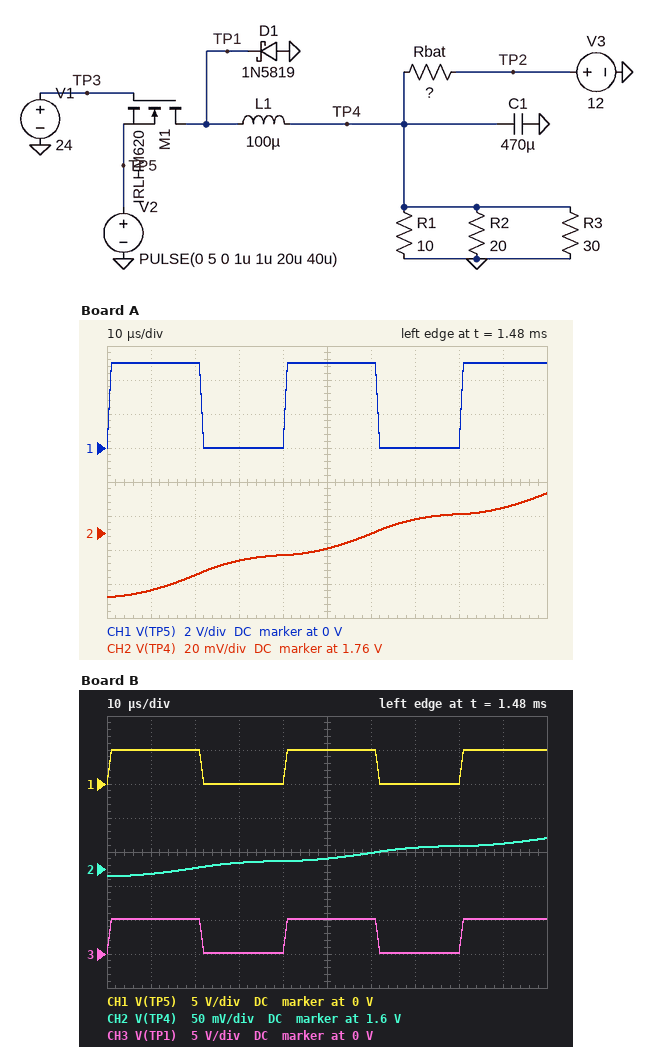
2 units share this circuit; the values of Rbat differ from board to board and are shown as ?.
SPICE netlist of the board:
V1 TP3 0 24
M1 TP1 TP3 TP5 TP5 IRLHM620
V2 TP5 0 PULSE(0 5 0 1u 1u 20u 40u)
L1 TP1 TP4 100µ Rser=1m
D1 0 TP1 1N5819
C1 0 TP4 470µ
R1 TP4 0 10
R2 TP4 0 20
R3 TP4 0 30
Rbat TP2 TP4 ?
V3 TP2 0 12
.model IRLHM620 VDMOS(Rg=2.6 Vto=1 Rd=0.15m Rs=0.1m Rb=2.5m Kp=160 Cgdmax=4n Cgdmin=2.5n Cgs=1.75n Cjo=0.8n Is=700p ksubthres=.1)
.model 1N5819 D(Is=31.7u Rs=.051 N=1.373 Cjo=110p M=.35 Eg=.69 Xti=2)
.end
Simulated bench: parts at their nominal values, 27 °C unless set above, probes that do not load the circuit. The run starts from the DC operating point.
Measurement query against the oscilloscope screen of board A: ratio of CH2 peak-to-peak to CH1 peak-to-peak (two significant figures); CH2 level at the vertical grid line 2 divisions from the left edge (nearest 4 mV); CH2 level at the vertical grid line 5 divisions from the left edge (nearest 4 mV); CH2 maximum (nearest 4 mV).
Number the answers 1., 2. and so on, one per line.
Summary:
1. 0.012
2. 1.736 V
3. 1.752 V
4. 1.784 V
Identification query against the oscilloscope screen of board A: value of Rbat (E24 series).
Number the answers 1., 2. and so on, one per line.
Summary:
1. 0.051 Ω
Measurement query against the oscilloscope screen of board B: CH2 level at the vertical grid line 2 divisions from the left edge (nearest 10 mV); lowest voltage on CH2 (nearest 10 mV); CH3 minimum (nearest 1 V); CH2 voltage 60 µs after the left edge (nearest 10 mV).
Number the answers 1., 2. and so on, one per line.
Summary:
1. 1.60 V
2. 1.59 V
3. 0 V
4. 1.62 V
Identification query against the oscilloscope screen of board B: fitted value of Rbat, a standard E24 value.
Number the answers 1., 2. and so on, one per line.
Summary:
1. 0.039 Ω
